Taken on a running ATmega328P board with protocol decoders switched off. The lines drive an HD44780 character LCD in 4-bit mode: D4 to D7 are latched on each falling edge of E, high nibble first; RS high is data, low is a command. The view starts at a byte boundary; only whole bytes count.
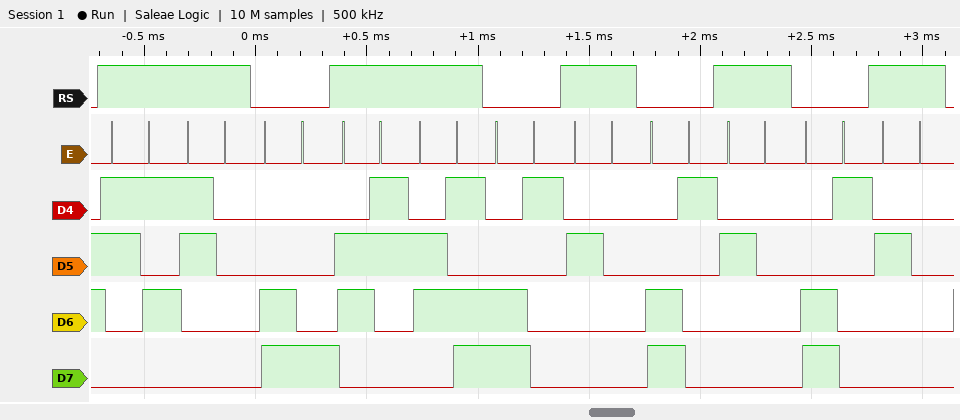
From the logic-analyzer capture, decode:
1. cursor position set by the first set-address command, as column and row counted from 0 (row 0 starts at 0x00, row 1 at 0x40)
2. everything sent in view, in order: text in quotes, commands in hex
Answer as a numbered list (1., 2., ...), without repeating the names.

1. column 8, row 1
2. "50" 0xC8 "cm" 0xC1 " " 0xC1 " " 0xC1 " "
